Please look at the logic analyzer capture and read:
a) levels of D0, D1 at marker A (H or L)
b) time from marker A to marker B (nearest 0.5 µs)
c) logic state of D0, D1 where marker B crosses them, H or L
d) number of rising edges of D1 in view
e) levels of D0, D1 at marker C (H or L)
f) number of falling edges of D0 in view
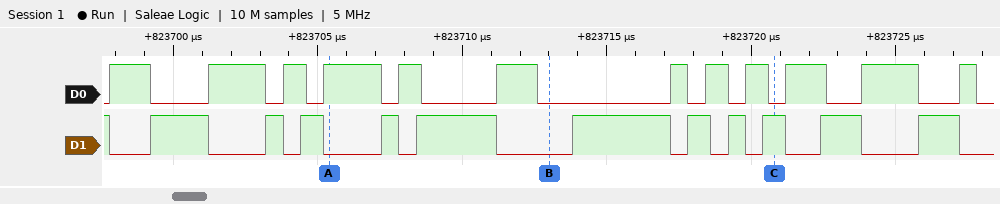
D0=H, D1=L
7.5 µs
D0=L, D1=L
11
D0=L, D1=H
12
